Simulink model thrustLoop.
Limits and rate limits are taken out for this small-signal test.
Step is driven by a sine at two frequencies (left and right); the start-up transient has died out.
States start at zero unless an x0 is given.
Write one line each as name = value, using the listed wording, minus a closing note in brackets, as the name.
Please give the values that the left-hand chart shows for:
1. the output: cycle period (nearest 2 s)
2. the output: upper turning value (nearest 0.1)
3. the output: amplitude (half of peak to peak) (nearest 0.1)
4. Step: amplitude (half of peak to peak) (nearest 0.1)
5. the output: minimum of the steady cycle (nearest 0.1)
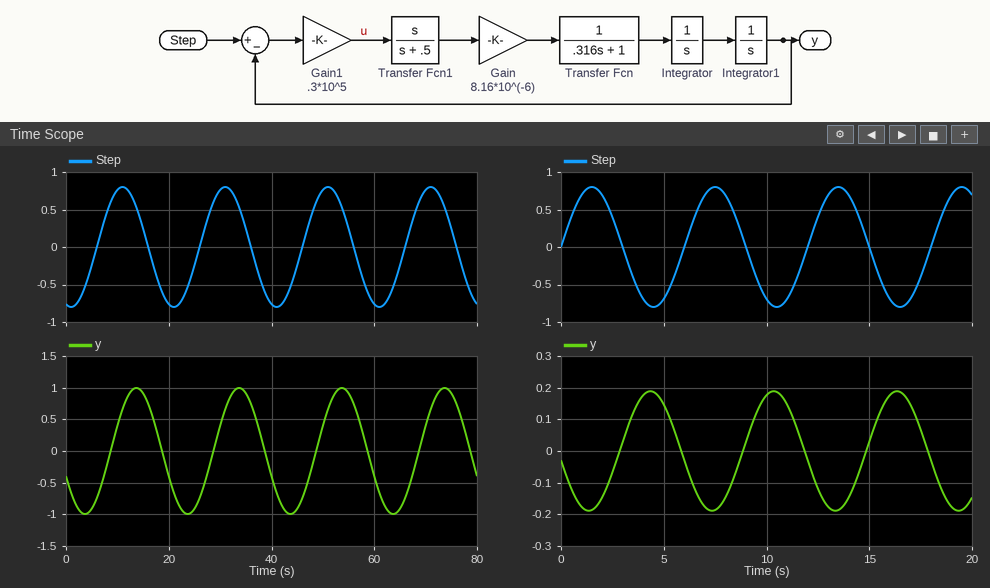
the output: cycle period = 20 s
the output: upper turning value = 1.0
the output: amplitude (half of peak to peak) = 1.0
Step: amplitude (half of peak to peak) = 0.8
the output: minimum of the steady cycle = -1.0
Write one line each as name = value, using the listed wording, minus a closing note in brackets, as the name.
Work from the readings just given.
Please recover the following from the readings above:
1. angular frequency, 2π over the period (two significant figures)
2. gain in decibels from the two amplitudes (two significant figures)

angular frequency, 2π over the period = 0.31 rad/s
gain in decibels from the two amplitudes = 1.9 dB
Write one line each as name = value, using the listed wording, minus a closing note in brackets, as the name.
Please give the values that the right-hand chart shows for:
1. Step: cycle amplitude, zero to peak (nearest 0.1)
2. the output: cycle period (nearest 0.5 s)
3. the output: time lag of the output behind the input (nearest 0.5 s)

Step: cycle amplitude, zero to peak = 0.8
the output: cycle period = 6.0 s
the output: time lag of the output behind the input = 3.0 s
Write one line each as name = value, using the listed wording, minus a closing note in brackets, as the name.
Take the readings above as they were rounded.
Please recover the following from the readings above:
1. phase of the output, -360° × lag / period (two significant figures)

phase of the output, -360° × lag / period = -180°
